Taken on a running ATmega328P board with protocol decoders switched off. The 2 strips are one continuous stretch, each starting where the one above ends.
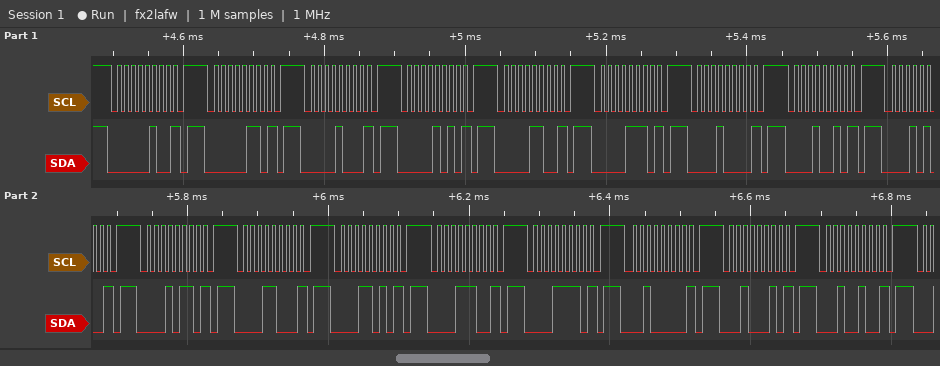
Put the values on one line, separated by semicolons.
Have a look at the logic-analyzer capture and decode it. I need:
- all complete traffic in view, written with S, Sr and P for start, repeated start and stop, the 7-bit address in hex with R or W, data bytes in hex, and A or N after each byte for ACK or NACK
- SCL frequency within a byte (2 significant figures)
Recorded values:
S 02W N P S 03W N P S 04W N P S 05W N P S 06W N P S 07W N P S 08W N P S 09W N P S 0AW N P S 0BW N P S 0CW N P S 0DW N P S 0EW N P S 0FW N P S 10W N P S 11W N P S 12W N P; 100 kHz
